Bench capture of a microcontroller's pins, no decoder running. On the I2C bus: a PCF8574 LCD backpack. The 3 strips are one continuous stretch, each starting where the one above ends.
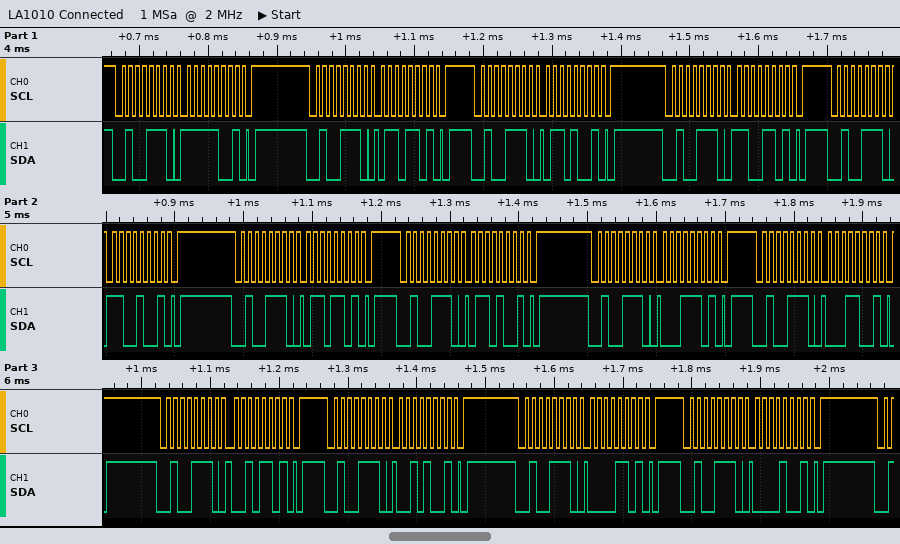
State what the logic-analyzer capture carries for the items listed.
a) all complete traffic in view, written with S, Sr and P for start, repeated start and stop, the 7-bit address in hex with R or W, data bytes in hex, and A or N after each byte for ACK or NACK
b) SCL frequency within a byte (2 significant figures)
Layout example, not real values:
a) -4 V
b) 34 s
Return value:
a) S 27W A F9 A P S 27W A 6D A P S 27W A 69 A P S 27W A CD A P S 27W A C9 A P S 27W A 6D A P S 27W A 69 A P S 27W A 1D A P S 27W A 19 A P S 27W A 2D A P S 27W A 29 A P S 27W A 0D A P S 27W A 09 A P
b) 100 kHz
